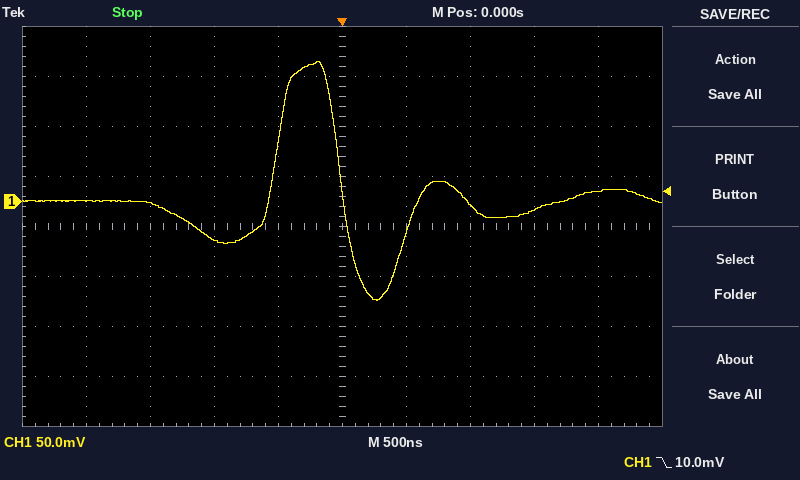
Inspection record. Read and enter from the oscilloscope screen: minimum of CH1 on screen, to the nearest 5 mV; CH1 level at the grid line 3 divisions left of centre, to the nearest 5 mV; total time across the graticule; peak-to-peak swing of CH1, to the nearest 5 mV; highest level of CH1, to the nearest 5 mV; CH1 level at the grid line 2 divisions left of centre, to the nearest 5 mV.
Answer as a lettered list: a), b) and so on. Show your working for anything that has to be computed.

a) -100 mV
b) 0 mV
c) 5 µs
d) 140 mV − (-100 mV) = 240 mV
e) 140 mV
f) -40 mV
